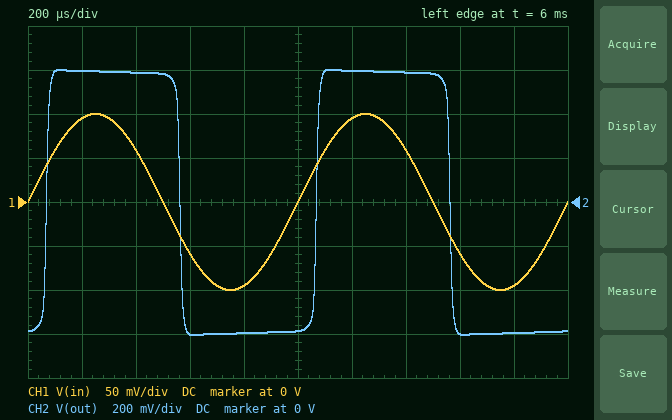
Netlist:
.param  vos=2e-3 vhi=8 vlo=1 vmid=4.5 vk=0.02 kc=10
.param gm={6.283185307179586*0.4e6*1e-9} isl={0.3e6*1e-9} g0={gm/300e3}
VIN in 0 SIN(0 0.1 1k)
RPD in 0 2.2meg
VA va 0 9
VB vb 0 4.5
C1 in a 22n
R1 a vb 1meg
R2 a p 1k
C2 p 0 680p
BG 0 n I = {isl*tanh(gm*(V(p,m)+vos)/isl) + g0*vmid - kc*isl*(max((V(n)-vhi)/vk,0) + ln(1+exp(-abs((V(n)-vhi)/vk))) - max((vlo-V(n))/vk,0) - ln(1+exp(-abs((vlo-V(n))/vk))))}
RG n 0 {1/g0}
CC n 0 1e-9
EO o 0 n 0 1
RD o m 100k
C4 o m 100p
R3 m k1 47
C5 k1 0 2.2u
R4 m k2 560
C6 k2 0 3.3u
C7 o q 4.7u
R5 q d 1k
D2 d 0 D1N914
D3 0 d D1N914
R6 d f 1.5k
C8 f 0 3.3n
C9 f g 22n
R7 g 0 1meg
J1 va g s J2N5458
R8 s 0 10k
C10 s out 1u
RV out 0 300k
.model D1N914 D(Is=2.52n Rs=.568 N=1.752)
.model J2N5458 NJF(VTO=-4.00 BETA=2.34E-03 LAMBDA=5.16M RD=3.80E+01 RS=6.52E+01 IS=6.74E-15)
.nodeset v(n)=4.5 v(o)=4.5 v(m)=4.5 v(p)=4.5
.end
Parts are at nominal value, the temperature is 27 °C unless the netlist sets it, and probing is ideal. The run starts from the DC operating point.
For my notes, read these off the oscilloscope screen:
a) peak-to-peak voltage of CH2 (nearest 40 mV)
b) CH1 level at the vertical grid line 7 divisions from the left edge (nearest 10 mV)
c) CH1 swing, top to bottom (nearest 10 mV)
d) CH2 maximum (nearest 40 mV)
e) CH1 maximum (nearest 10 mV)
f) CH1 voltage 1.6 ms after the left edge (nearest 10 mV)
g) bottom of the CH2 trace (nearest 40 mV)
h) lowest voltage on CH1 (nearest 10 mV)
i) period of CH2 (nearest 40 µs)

1.20 V
60 mV
200 mV
600 mV
100 mV
-60 mV
-600 mV
-100 mV
1.00 ms
